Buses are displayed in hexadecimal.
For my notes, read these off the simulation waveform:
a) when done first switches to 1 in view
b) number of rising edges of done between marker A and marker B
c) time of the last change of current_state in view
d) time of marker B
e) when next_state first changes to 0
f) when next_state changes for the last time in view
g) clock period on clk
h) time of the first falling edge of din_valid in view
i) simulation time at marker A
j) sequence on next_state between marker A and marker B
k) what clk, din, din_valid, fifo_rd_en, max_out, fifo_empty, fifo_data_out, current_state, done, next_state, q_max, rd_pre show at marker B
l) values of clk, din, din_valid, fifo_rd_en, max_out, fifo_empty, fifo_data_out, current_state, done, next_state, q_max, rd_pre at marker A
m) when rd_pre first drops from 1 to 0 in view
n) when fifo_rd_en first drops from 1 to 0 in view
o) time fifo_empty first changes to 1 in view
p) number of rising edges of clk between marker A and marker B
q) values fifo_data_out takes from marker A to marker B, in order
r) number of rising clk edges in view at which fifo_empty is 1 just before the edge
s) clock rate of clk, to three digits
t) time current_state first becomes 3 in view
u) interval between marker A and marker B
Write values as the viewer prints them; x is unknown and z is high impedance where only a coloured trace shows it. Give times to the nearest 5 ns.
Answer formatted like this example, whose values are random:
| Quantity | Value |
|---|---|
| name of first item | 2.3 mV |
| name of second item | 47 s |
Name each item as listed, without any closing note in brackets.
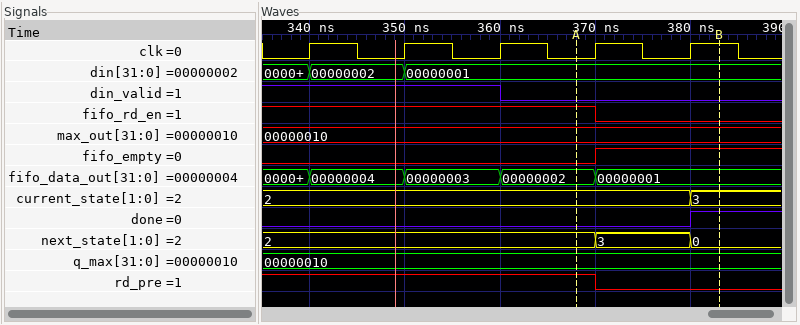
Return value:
| Quantity | Value |
|---|---|
| when done first switches to 1 in view | 380 ns |
| number of rising edges of done between marker A and marker B | 1 |
| time of the last change of current_state in view | 380 ns |
| time of marker B | 385 ns |
| when next_state first changes to 0 | 380 ns |
| when next_state changes for the last time in view | 380 ns |
| clock period on clk | 10 ns |
| time of the first falling edge of din_valid in view | 360 ns |
| simulation time at marker A | 370 ns |
| sequence on next_state between marker A and marker B | 2, 3, 0 |
| what clk, din, din_valid, fifo_rd_en, max_out, fifo_empty, fifo_data_out, current_state, done, next_state, q_max, rd_pre show at marker B | clk=1, din=00000001, din_valid=0, fifo_rd_en=0, max_out=00000010, fifo_empty=1, fifo_data_out=00000001, current_state=3, done=1, next_state=0, q_max=00000010, rd_pre=0 |
| values of clk, din, din_valid, fifo_rd_en, max_out, fifo_empty, fifo_data_out, current_state, done, next_state, q_max, rd_pre at marker A | clk=0, din=00000001, din_valid=0, fifo_rd_en=1, max_out=00000010, fifo_empty=0, fifo_data_out=00000002, current_state=2, done=0, next_state=2, q_max=00000010, rd_pre=1 |
| when rd_pre first drops from 1 to 0 in view | 370 ns |
| when fifo_rd_en first drops from 1 to 0 in view | 370 ns |
| time fifo_empty first changes to 1 in view | 370 ns |
| number of rising edges of clk between marker A and marker B | 2 |
| values fifo_data_out takes from marker A to marker B, in order | 00000002, 00000001 |
| number of rising clk edges in view at which fifo_empty is 1 just before the edge | 1 |
| clock rate of clk, to three digits | 100 MHz |
| time current_state first becomes 3 in view | 380 ns |
| interval between marker A and marker B | 15 ns |
